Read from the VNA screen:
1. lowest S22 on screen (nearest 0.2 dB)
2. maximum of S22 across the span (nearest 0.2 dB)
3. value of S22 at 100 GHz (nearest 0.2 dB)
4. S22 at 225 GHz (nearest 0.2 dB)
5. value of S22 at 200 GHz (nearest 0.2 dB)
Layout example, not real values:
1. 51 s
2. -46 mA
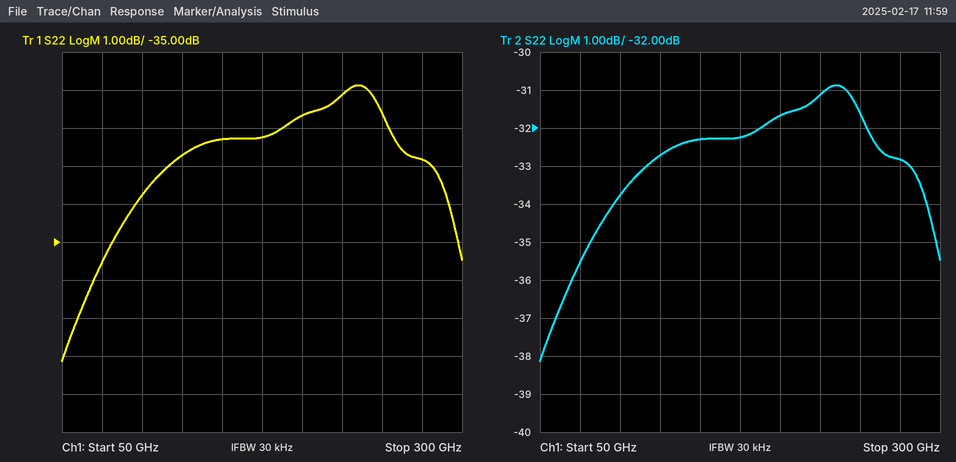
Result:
1. -38.2 dB
2. -30.8 dB
3. -33.8 dB
4. -31.2 dB
5. -31.6 dB
